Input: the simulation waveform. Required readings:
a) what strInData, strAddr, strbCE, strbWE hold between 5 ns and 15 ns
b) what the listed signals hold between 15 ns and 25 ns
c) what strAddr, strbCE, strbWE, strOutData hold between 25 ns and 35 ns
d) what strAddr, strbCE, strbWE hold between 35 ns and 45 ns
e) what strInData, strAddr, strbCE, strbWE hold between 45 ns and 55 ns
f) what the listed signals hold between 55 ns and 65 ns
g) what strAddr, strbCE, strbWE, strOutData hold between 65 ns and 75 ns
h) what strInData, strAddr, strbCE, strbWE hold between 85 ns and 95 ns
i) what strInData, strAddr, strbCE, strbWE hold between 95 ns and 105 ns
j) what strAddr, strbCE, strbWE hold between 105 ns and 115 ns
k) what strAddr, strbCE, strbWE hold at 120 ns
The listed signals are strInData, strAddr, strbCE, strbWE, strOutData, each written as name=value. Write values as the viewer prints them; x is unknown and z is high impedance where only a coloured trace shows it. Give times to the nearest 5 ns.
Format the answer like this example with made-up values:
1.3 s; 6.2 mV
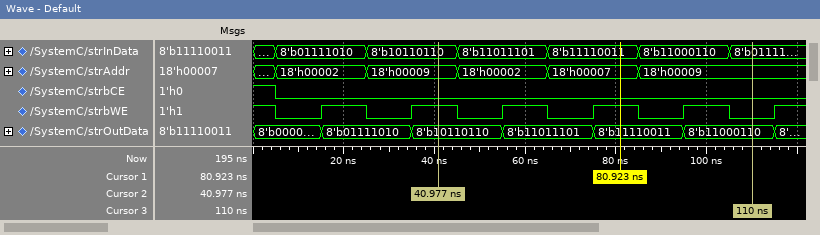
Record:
strInData=8'b01111010, strAddr=18'h00002, strbCE=0, strbWE=0; strInData=8'b01111010, strAddr=18'h00002, strbCE=0, strbWE=1, strOutData=8'b01111010; strAddr=18'h00009, strbCE=0, strbWE=0, strOutData=8'b01111010; strAddr=18'h00009, strbCE=0, strbWE=1; strInData=8'b11011101, strAddr=18'h00002, strbCE=0, strbWE=0; strInData=8'b11011101, strAddr=18'h00002, strbCE=0, strbWE=1, strOutData=8'b11011101; strAddr=18'h00007, strbCE=0, strbWE=0, strOutData=8'b11011101; strInData=8'b11000110, strAddr=18'h00009, strbCE=0, strbWE=0; strInData=8'b11000110, strAddr=18'h00009, strbCE=0, strbWE=1; strAddr=18'h00009, strbCE=0, strbWE=0; strAddr=18'h00009, strbCE=0, strbWE=1
